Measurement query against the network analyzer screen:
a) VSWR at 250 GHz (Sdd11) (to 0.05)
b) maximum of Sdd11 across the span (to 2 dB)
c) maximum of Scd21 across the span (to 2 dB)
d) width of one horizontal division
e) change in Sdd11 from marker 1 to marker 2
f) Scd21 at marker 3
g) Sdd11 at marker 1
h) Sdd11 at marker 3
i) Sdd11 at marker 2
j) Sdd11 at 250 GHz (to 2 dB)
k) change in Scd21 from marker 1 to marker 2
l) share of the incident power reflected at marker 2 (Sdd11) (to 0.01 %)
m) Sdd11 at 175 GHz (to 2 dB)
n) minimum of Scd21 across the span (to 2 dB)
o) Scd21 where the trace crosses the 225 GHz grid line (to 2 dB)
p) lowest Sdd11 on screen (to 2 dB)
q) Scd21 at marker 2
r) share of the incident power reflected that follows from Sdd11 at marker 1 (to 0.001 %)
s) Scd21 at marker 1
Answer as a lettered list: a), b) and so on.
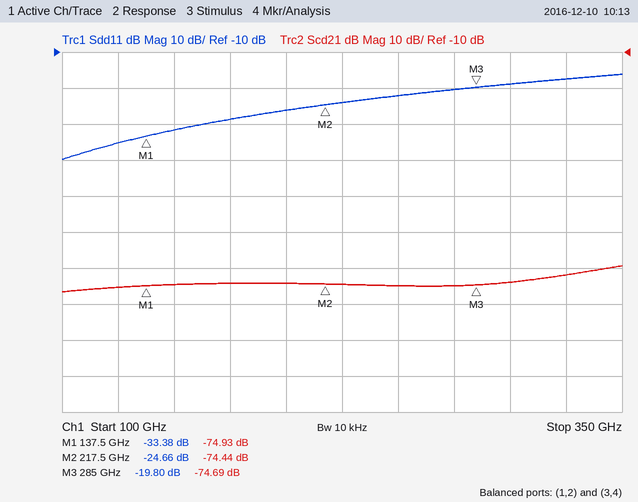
a) 1.15
b) -16 dB
c) -70 dB
d) 25 GHz
e) 8.72 dB
f) -74.69 dB
g) -33.38 dB
h) -19.80 dB
i) -24.66 dB
j) -22 dB
k) 0.49 dB
l) 0.34 %
m) -28 dB
n) -76 dB
o) -74 dB
p) -40 dB
q) -74.44 dB
r) 0.046 %
s) -74.93 dB
